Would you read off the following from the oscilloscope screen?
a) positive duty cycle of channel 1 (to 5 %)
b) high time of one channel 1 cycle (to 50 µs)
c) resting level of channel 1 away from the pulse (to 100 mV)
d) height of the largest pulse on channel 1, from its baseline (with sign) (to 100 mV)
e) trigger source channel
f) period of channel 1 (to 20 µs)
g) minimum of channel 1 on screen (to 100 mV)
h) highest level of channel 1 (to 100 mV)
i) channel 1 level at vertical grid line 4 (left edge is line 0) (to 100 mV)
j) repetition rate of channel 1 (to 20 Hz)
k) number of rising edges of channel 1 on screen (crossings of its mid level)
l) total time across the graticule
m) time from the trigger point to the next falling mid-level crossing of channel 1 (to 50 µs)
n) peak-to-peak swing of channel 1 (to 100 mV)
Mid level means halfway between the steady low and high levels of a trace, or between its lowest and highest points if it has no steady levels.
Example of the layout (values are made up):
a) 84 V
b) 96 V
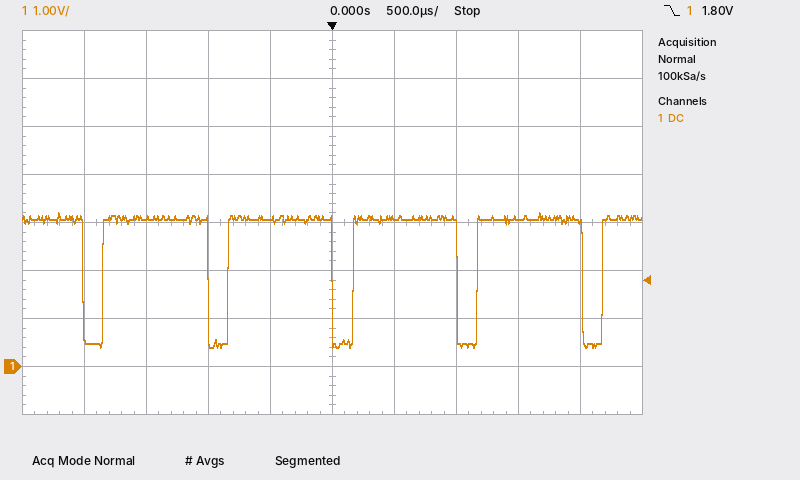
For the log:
a) 85 %
b) 850 µs
c) 3.1 V
d) -2.7 V
e) channel 1
f) 1.00 ms
g) 400 mV
h) 3.2 V
i) 3.1 V
j) 1.00 kHz
k) 5
l) 5 ms
m) 1.00 ms
n) 2.8 V
